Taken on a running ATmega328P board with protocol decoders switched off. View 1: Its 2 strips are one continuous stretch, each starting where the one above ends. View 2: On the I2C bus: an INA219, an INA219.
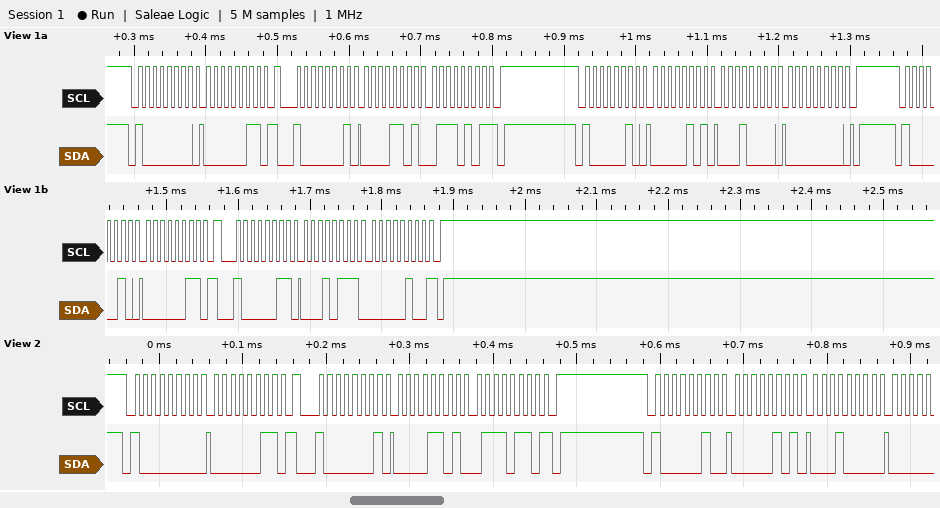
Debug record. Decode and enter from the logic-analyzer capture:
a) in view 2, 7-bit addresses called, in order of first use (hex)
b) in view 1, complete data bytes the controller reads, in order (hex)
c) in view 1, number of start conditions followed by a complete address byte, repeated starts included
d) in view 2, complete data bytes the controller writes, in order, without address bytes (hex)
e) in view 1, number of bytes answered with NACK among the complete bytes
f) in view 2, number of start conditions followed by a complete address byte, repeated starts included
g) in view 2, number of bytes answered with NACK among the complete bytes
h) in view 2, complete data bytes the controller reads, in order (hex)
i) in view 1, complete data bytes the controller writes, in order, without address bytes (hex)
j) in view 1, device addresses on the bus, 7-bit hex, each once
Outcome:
0x40 0x41
0D 75 17 04
5
03 05 10
2
3
1
0D 76
03 05 10 00 03
0x40 0x41
